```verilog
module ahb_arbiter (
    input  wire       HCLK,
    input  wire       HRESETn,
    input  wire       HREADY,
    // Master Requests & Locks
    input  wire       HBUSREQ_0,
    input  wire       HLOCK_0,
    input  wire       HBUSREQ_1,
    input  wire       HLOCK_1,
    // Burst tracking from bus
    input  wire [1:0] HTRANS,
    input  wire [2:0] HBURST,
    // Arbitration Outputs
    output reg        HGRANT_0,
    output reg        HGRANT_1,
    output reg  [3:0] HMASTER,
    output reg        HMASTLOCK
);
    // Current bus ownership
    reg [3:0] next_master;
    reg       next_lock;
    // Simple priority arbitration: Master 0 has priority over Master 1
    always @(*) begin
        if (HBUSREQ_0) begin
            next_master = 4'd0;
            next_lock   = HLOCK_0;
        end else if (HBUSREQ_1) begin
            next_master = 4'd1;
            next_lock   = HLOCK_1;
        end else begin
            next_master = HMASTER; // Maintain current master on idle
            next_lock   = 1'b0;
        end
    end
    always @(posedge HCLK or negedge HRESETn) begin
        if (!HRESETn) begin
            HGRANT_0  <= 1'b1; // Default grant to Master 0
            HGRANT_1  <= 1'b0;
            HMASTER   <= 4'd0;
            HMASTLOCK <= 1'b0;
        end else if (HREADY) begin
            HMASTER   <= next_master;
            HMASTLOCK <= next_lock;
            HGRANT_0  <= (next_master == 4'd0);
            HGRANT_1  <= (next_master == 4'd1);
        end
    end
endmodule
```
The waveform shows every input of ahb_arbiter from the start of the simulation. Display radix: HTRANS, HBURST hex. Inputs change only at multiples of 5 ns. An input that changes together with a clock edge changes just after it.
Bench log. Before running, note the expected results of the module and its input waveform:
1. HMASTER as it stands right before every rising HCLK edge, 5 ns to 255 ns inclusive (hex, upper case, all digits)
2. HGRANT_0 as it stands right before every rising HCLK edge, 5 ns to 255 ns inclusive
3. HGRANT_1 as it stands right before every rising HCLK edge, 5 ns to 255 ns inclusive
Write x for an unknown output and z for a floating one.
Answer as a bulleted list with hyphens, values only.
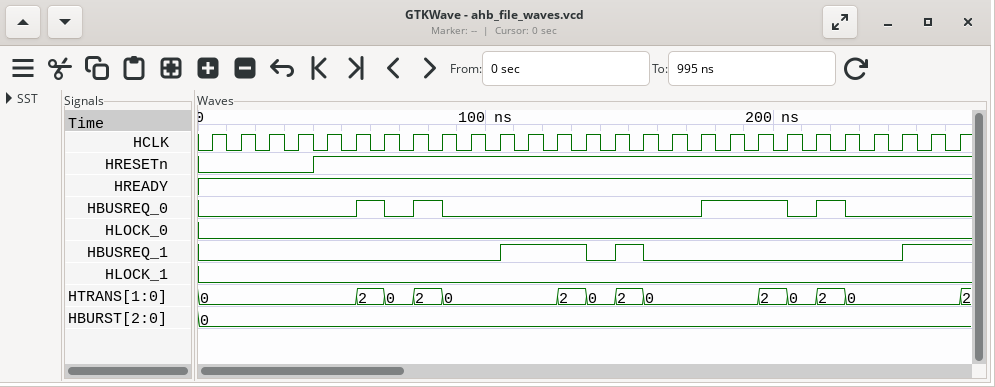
- 0, 0, 0, 0, 0, 0, 0, 0, 0, 0, 0, 0, 1, 1, 1, 1, 1, 1, 1, 0, 0, 0, 0, 0, 0, 0
- 1 1 1 1 1 1 1 1 1 1 1 1 0 0 0 0 0 0 0 1 1 1 1 1 1 1
- 0 0 0 0 0 0 0 0 0 0 0 0 1 1 1 1 1 1 1 0 0 0 0 0 0 0
